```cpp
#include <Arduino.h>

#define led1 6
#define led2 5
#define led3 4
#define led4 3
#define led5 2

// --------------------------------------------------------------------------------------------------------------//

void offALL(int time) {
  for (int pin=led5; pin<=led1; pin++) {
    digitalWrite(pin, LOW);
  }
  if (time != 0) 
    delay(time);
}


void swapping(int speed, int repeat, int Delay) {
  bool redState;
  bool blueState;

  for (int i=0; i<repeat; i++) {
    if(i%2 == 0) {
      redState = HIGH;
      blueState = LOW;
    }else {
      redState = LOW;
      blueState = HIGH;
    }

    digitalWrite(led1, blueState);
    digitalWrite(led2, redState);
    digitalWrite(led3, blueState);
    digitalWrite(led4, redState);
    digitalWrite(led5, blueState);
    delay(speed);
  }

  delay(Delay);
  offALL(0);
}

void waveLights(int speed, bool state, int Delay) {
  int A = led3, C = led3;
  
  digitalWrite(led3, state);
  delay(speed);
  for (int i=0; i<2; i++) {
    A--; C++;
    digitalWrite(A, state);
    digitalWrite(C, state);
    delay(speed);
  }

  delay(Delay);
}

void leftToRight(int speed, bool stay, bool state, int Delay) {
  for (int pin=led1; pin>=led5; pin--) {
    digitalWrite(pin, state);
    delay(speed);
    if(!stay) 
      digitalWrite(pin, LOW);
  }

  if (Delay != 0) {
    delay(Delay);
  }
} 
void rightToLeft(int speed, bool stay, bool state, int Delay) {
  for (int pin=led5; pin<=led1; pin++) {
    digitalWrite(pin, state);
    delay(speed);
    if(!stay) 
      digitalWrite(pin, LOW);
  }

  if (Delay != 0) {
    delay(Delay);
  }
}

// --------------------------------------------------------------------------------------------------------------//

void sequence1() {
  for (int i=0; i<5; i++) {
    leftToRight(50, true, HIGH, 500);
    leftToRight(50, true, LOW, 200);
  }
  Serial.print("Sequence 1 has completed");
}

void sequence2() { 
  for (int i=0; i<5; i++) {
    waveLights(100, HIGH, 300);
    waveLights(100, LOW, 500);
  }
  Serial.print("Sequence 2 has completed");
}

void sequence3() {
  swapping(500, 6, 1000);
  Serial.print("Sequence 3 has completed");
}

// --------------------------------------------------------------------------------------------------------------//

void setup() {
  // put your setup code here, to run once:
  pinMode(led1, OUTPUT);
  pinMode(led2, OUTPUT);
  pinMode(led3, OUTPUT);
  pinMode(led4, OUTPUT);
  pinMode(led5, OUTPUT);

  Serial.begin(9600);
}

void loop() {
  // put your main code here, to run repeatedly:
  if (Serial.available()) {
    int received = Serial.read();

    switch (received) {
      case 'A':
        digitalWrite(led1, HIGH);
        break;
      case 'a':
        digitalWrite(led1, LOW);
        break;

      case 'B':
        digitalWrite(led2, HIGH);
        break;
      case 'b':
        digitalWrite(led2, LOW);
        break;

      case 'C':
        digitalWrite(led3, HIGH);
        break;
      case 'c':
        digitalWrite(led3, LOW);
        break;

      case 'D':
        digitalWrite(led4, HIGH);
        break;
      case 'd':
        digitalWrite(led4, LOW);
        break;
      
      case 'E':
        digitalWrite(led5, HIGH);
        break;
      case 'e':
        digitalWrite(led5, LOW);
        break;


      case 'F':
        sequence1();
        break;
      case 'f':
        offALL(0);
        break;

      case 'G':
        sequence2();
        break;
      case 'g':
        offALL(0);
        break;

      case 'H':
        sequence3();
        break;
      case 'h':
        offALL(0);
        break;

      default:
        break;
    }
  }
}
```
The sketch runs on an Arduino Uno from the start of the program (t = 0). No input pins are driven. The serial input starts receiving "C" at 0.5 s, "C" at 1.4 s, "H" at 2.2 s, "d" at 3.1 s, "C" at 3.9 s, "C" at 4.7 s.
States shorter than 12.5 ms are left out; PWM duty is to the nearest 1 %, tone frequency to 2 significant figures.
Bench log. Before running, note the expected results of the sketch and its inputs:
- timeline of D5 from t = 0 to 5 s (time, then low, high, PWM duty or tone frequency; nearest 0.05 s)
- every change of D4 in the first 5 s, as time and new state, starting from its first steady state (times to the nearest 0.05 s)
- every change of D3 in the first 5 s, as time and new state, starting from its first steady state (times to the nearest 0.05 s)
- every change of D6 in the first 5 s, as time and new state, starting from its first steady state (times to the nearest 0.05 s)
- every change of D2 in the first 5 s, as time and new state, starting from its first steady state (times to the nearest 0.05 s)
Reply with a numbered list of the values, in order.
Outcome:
1. 0 s low; 2.2 s high; 2.7 s low; 3.2 s high; 3.7 s low; 4.2 s high; 4.7 s low
2. 0 s low; 0.5 s high; 2.2 s low; 2.7 s high; 3.2 s low; 3.7 s high; 4.2 s low; 4.7 s high
3. 0 s low; 2.2 s high; 2.7 s low; 3.2 s high; 3.7 s low; 4.2 s high; 4.7 s low
4. 0 s low; 2.7 s high; 3.2 s low; 3.7 s high; 4.2 s low; 4.7 s high
5. 0 s low; 2.7 s high; 3.2 s low; 3.7 s high; 4.2 s low; 4.7 s high
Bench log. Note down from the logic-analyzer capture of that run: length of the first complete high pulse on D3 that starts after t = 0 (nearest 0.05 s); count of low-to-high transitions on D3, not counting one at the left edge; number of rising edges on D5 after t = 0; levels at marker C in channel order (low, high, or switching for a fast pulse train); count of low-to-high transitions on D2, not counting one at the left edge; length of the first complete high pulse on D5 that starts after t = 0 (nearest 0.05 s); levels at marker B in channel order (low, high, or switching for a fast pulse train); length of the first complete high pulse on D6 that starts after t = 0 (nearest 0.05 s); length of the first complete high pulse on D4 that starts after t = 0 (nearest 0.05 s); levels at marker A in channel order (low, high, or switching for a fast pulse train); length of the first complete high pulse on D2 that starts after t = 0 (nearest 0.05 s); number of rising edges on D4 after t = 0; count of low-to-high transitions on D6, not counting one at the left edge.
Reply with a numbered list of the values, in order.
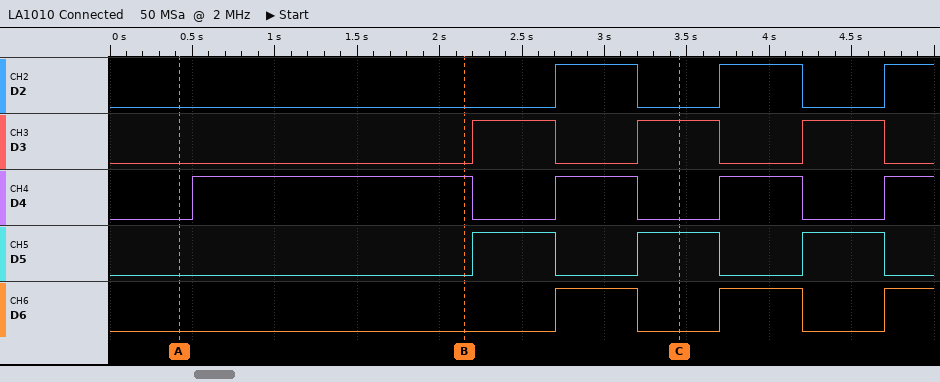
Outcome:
1. 0.50 s
2. 3
3. 3
4. D2 low, D3 high, D4 low, D5 high, D6 low
5. 3
6. 0.50 s
7. D2 low, D3 low, D4 high, D5 low, D6 low
8. 0.50 s
9. 1.70 s
10. D2 low, D3 low, D4 low, D5 low, D6 low
11. 0.50 s
12. 4
13. 3
